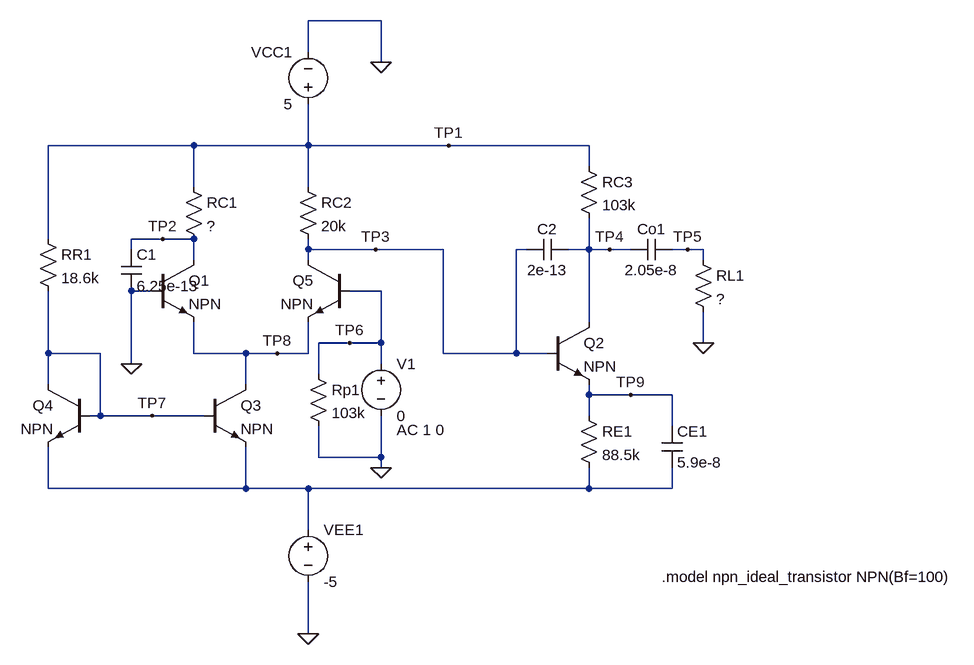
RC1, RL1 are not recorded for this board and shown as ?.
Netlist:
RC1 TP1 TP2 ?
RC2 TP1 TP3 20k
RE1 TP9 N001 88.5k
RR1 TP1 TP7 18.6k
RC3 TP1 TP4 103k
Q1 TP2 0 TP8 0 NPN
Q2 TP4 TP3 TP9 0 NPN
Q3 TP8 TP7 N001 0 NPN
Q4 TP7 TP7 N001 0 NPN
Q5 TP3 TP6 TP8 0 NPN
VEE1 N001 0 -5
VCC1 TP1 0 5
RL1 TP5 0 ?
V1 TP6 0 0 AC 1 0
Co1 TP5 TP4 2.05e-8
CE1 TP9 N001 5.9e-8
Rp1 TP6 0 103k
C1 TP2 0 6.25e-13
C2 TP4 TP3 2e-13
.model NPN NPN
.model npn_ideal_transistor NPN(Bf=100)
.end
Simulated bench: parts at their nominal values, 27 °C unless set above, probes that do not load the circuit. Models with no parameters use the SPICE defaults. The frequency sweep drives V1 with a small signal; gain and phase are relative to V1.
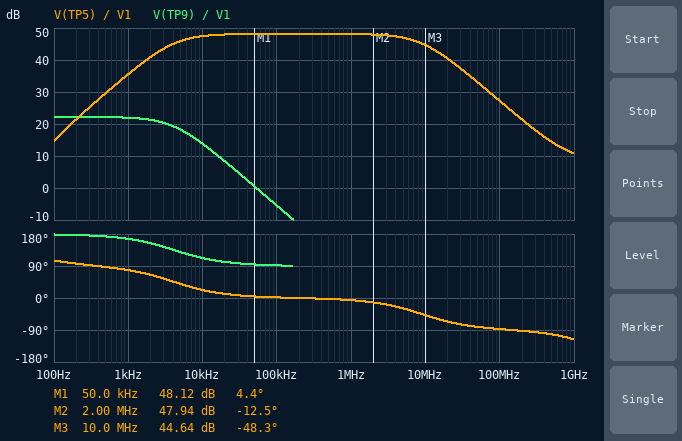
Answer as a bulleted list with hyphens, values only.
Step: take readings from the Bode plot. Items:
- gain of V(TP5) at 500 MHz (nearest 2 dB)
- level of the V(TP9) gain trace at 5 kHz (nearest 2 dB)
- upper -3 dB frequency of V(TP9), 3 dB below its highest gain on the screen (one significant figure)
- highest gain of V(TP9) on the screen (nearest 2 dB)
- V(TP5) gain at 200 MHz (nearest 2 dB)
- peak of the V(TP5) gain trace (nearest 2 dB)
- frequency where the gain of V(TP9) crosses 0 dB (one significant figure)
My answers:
- 14 dB
- 18 dB
- 4 kHz
- 22 dB
- 22 dB
- 48 dB
- 50 kHz
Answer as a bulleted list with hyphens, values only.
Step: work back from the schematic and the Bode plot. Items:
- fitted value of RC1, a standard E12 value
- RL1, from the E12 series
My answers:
- 56 kΩ
- 15 kΩ
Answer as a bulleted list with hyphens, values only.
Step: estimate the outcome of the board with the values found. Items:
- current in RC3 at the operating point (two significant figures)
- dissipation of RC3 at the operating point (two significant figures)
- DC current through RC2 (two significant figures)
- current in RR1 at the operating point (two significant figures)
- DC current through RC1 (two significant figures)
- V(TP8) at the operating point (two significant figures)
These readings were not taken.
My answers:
- 41 µA
- 170 µW
- 280 µA
- 500 µA
- 100 µA
- -740 mV
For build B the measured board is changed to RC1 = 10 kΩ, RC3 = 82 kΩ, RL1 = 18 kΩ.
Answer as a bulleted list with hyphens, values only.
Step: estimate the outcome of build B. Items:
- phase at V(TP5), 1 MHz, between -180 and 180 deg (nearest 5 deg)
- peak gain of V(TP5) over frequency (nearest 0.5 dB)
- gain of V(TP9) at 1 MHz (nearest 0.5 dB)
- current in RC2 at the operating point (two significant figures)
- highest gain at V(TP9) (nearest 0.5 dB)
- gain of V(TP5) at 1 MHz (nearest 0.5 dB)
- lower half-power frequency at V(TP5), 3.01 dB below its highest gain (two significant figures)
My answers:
- -30 deg
- 65.5 dB
- -10.0 dB
- 240 µA
- 39.5 dB
- 64.5 dB
- 3.8 kHz
